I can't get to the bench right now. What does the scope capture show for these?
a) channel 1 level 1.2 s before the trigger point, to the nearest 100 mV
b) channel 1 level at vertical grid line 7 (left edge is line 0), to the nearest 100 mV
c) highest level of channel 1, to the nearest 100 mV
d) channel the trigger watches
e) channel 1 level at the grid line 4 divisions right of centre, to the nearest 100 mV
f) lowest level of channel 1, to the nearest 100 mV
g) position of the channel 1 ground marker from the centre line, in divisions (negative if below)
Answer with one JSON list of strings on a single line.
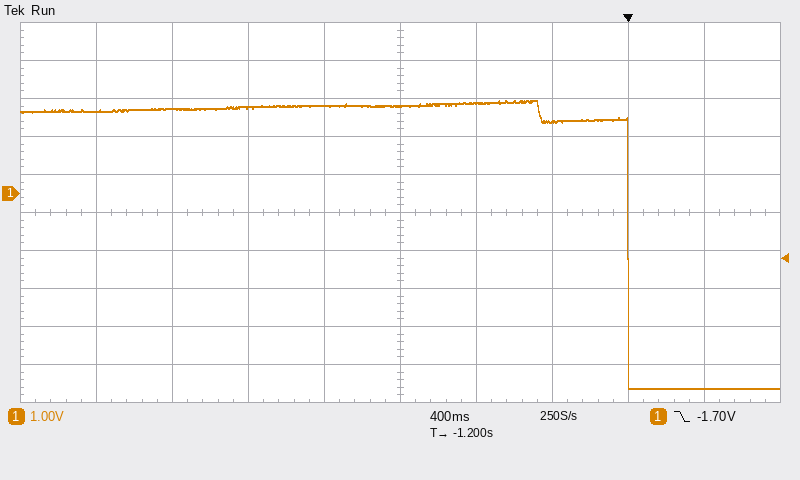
["2.3 V", "1.9 V", "2.4 V", "channel 1", "-5.1 V", "-5.1 V", "+0.5 div"]
